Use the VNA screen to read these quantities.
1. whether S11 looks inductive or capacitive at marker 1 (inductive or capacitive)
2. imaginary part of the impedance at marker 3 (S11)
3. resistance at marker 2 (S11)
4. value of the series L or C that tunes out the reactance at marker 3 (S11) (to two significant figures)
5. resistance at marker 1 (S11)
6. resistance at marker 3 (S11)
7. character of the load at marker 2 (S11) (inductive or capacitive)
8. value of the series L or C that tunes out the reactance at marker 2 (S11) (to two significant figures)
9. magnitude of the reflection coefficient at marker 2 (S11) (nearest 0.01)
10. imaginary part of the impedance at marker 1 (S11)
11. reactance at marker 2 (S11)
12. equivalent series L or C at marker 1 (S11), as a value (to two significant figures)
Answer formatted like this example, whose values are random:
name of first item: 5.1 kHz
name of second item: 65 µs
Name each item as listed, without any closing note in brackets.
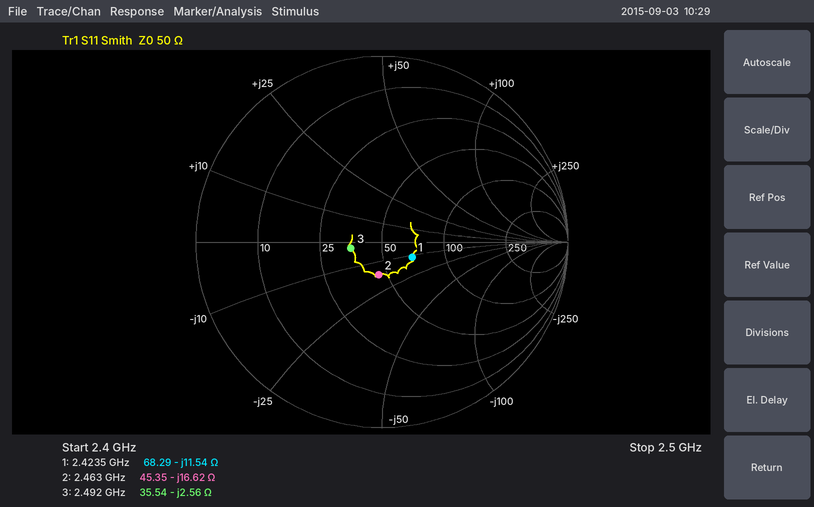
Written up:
whether S11 looks inductive or capacitive at marker 1: capacitive
imaginary part of the impedance at marker 3: -2.56 Ω
resistance at marker 2: 45.35 Ω
value of the series L or C that tunes out the reactance at marker 3 (S11): 160 pH
resistance at marker 1: 68.29 Ω
resistance at marker 3: 35.54 Ω
character of the load at marker 2 (S11): capacitive
value of the series L or C that tunes out the reactance at marker 2 (S11): 1.1 nH
magnitude of the reflection coefficient at marker 2 (S11): 0.18
imaginary part of the impedance at marker 1: -11.54 Ω
reactance at marker 2: -16.62 Ω
equivalent series L or C at marker 1 (S11), as a value: 5.7 pF
